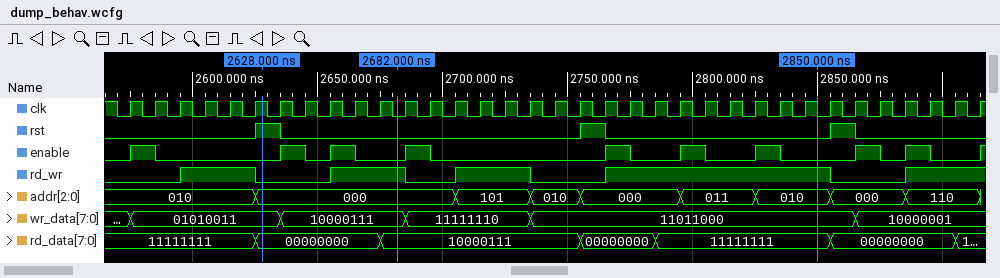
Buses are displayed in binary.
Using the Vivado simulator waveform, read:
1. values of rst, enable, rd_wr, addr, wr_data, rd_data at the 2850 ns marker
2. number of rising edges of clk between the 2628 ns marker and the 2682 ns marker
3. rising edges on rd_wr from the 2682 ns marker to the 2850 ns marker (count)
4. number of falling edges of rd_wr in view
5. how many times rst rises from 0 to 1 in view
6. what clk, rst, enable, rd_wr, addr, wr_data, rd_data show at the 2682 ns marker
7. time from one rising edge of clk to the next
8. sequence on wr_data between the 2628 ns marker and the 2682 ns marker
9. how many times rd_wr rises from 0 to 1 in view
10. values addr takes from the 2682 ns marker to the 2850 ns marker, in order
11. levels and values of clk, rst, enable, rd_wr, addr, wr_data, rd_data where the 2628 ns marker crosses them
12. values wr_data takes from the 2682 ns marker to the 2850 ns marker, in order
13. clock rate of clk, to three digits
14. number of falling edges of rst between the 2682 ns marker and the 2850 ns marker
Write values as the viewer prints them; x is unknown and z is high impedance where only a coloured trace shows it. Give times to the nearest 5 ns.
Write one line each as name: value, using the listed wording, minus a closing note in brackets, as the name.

values of rst, enable, rd_wr, addr, wr_data, rd_data at the 2850 ns marker: rst=0, enable=0, rd_wr=1, addr=010, wr_data=11011000, rd_data=11111111
number of rising edges of clk between the 2628 ns marker and the 2682 ns marker: 5
rising edges on rd_wr from the 2682 ns marker to the 2850 ns marker: 2
number of falling edges of rd_wr in view: 4
how many times rst rises from 0 to 1 in view: 3
what clk, rst, enable, rd_wr, addr, wr_data, rd_data show at the 2682 ns marker: clk=0, rst=0, enable=0, rd_wr=1, addr=000, wr_data=10000111, rd_data=10000111
time from one rising edge of clk to the next: 10 ns
sequence on wr_data between the 2628 ns marker and the 2682 ns marker: 01010011, 10000111
how many times rd_wr rises from 0 to 1 in view: 5
values addr takes from the 2682 ns marker to the 2850 ns marker, in order: 000, 101, 010, 000, 011, 010
levels and values of clk, rst, enable, rd_wr, addr, wr_data, rd_data where the 2628 ns marker crosses them: clk=1, rst=1, enable=0, rd_wr=0, addr=000, wr_data=01010011, rd_data=00000000
values wr_data takes from the 2682 ns marker to the 2850 ns marker, in order: 10000111, 11111110, 11011000
clock rate of clk, to three digits: 100 MHz
number of falling edges of rst between the 2682 ns marker and the 2850 ns marker: 1
